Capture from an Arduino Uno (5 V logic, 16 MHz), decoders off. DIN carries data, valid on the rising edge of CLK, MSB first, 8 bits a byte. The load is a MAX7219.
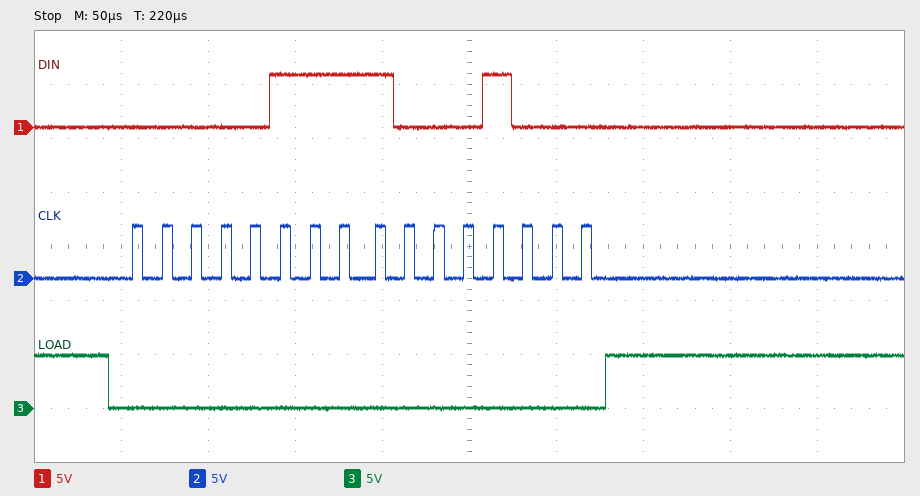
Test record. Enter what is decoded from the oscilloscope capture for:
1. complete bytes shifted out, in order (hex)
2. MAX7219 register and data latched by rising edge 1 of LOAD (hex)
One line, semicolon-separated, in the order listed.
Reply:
07 88; register 0x7, data 0x88
